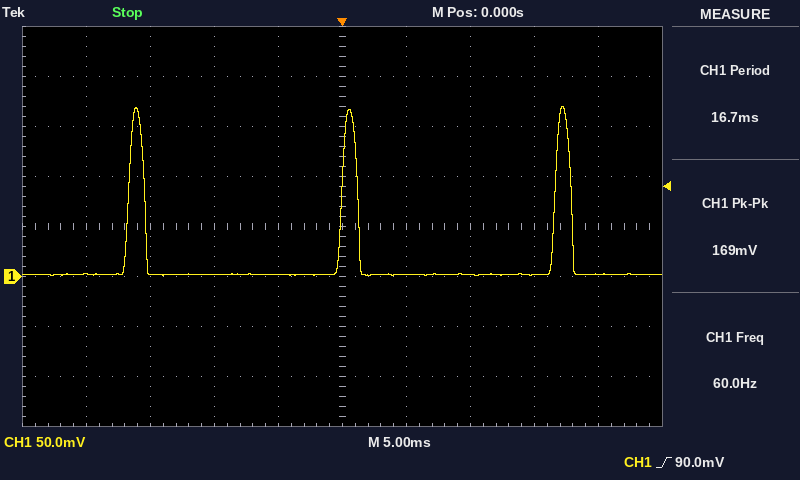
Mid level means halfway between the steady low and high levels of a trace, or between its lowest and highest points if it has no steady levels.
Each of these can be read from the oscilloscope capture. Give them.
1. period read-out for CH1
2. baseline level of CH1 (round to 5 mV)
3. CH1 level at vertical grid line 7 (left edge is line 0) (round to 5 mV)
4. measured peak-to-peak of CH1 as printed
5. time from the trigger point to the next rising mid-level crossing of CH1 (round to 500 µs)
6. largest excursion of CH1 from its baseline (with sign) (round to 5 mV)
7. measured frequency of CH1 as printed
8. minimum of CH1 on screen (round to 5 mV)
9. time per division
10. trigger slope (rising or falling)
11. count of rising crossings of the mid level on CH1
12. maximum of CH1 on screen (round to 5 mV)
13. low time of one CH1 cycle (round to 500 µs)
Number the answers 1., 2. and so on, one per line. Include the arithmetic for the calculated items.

1. 16.7 ms
2. 0 mV
3. 0 mV
4. 169 mV
5. 16.5 ms
6. 170 mV − (0 mV) = +170 mV
7. 60.0 Hz
8. 0 mV
9. 5 ms
10. rising
11. 3
12. 170 mV
13. 15.5 ms
